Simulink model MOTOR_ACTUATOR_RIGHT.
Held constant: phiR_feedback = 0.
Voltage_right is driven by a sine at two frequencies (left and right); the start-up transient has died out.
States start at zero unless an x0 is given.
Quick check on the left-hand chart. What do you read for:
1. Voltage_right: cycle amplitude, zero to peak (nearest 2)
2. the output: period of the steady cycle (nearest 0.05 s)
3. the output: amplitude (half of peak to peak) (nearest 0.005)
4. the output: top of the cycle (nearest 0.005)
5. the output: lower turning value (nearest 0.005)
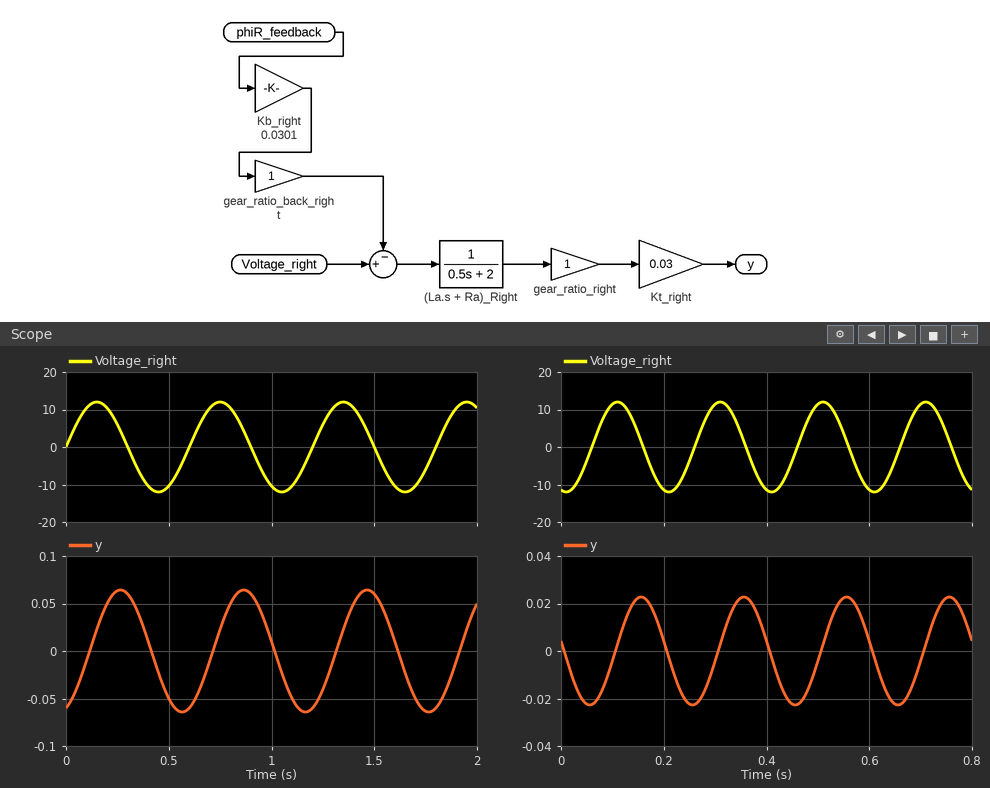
12
0.60 s
0.065
0.065
-0.065
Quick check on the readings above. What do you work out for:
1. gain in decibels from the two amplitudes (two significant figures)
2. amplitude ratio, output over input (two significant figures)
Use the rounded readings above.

-45 dB
0.0054
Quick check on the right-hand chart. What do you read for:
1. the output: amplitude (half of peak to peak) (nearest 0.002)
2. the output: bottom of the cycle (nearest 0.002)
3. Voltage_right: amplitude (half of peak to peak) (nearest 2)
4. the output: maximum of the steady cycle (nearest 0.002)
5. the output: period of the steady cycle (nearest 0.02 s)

0.022
-0.022
12
0.022
0.20 s
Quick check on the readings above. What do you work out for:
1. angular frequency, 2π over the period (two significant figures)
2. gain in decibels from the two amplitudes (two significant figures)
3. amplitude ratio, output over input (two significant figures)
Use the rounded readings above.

31 rad/s
-55 dB
0.0018
